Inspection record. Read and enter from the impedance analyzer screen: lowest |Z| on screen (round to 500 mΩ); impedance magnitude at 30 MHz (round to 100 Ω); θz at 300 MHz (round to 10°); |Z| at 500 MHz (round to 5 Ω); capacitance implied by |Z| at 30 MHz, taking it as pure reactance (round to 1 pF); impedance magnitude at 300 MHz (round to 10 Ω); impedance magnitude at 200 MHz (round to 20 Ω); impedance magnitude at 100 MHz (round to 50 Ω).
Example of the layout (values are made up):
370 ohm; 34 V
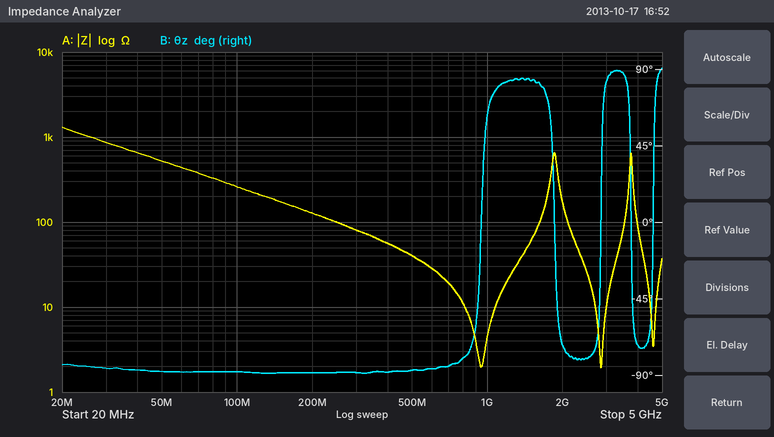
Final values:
2.0 Ω; 900 Ω; -90°; 40 Ω; 6 pF; 80 Ω; 120 Ω; 250 Ω
